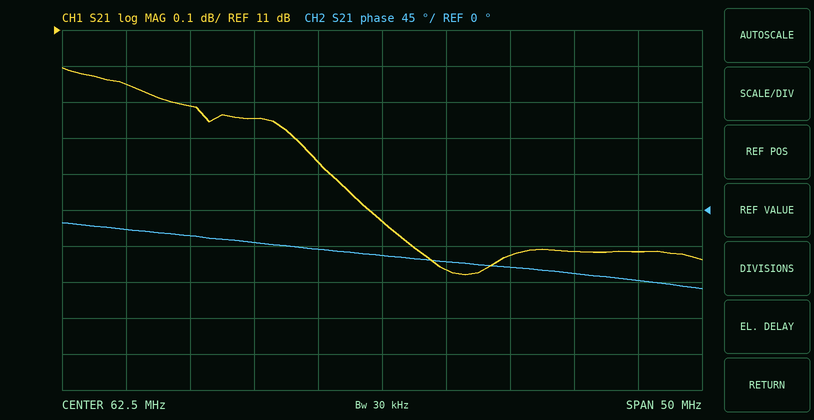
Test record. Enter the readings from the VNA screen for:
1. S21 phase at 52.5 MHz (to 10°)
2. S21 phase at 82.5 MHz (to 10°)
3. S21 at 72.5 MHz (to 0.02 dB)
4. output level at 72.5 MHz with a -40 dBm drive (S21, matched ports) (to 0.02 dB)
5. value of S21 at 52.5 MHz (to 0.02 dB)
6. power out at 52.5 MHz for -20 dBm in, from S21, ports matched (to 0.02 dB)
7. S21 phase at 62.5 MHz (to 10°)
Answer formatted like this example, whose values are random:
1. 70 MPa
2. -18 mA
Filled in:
1. -40°
2. -90°
3. 10.38 dB
4. -29.62 dBm
5. 10.76 dB
6. -9.24 dBm
7. -60°
